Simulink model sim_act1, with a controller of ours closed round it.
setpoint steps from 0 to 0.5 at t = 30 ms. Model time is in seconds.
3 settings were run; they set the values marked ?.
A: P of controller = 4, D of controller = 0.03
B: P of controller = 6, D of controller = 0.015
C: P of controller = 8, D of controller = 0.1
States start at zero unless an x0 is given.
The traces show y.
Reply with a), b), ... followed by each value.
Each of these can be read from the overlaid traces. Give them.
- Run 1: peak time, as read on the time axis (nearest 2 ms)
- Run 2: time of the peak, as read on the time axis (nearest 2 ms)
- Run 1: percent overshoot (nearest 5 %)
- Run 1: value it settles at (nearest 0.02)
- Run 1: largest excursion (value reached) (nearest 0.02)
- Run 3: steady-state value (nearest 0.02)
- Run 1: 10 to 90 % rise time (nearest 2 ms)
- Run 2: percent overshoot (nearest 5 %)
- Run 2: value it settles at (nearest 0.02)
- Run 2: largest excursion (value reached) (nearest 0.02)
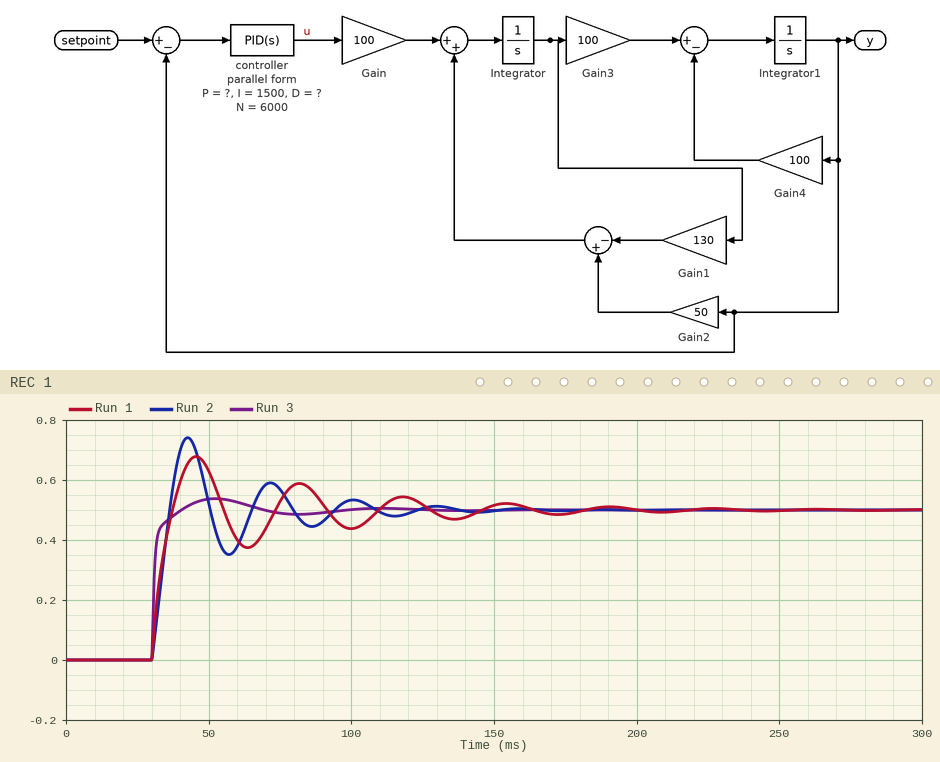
a) 46 ms
b) 42 ms
c) 35 %
d) 0.50
e) 0.68
f) 0.50
g) 6 ms
h) 50 %
i) 0.50
j) 0.74
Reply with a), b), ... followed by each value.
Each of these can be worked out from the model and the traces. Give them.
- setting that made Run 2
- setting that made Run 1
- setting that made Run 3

a) B
b) A
c) C
